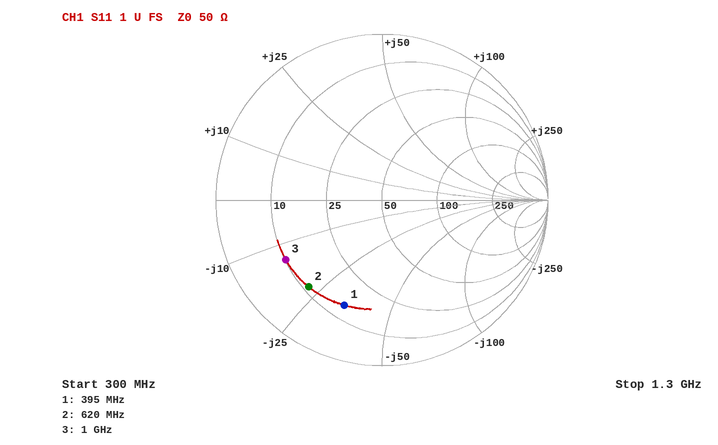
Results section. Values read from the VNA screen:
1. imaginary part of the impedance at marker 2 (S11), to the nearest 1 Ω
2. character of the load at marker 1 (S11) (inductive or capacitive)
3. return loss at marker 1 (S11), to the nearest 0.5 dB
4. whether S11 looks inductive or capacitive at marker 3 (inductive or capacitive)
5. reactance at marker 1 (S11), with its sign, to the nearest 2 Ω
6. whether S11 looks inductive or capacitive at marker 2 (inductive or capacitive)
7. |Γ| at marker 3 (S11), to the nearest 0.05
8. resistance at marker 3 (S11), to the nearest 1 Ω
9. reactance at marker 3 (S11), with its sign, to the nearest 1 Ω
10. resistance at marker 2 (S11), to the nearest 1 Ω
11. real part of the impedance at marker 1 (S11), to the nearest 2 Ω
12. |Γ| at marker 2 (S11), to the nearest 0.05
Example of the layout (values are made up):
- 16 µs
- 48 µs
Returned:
- -22 Ω
- capacitive
- 3.5 dB
- capacitive
- -34 Ω
- capacitive
- 0.70
- 10 Ω
- -14 Ω
- 11 Ω
- 14 Ω
- 0.70
